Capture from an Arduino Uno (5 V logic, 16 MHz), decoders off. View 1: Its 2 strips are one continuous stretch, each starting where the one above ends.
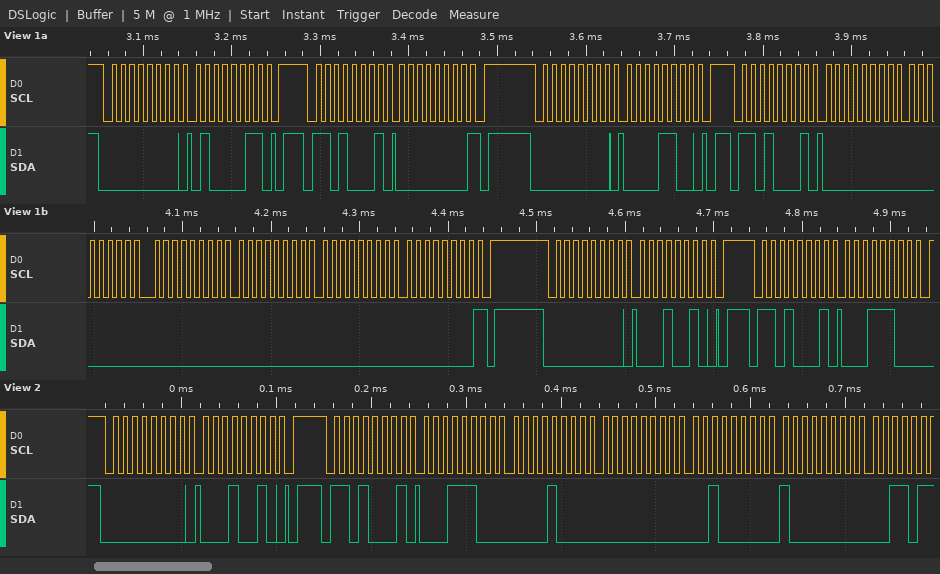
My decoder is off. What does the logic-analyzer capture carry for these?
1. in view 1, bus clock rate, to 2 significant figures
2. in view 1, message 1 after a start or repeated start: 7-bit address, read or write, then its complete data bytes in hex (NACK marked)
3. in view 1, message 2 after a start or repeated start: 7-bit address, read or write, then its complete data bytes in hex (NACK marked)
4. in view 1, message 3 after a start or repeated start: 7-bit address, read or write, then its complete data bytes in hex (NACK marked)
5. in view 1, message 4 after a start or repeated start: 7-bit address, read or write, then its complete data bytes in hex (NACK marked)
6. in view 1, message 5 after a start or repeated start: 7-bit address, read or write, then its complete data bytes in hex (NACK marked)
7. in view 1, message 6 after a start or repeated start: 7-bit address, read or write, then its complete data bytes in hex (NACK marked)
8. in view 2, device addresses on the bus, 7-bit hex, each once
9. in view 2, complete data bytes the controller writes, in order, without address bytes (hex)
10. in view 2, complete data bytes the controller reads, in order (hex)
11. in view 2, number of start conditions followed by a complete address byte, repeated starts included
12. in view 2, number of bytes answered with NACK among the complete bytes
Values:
100 kHz
0x00 write: 43
0x68 read: 00 NACK
0x00 write: 0C
0x68 read: 00 00 00 00 00 00 NACK
0x00 write: 12
0x68 read: 1C
0x00 0x68
12
1C 08 00 20 80
2
0
